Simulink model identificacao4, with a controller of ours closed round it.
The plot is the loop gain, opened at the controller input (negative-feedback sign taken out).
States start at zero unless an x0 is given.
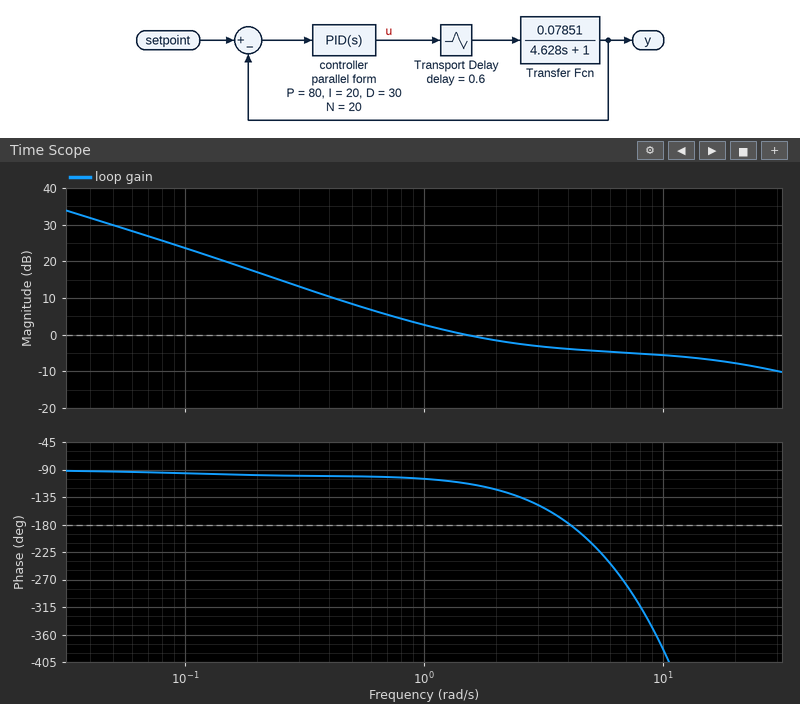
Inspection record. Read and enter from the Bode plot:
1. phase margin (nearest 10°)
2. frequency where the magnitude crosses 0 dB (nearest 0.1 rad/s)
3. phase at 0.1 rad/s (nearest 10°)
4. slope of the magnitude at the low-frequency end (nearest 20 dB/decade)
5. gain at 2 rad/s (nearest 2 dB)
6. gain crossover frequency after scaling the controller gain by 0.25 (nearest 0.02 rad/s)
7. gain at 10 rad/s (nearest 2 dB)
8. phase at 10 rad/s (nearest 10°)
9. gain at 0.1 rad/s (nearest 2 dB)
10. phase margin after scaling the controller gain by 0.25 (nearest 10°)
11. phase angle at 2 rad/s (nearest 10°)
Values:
70°
1.5 rad/s
-100°
-20 dB/decade
-2 dB
0.34 rad/s
-6 dB
-380°
24 dB
80°
-120°
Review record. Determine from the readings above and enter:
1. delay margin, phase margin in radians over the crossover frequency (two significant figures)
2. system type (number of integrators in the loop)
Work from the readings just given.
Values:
0.81 s
1
